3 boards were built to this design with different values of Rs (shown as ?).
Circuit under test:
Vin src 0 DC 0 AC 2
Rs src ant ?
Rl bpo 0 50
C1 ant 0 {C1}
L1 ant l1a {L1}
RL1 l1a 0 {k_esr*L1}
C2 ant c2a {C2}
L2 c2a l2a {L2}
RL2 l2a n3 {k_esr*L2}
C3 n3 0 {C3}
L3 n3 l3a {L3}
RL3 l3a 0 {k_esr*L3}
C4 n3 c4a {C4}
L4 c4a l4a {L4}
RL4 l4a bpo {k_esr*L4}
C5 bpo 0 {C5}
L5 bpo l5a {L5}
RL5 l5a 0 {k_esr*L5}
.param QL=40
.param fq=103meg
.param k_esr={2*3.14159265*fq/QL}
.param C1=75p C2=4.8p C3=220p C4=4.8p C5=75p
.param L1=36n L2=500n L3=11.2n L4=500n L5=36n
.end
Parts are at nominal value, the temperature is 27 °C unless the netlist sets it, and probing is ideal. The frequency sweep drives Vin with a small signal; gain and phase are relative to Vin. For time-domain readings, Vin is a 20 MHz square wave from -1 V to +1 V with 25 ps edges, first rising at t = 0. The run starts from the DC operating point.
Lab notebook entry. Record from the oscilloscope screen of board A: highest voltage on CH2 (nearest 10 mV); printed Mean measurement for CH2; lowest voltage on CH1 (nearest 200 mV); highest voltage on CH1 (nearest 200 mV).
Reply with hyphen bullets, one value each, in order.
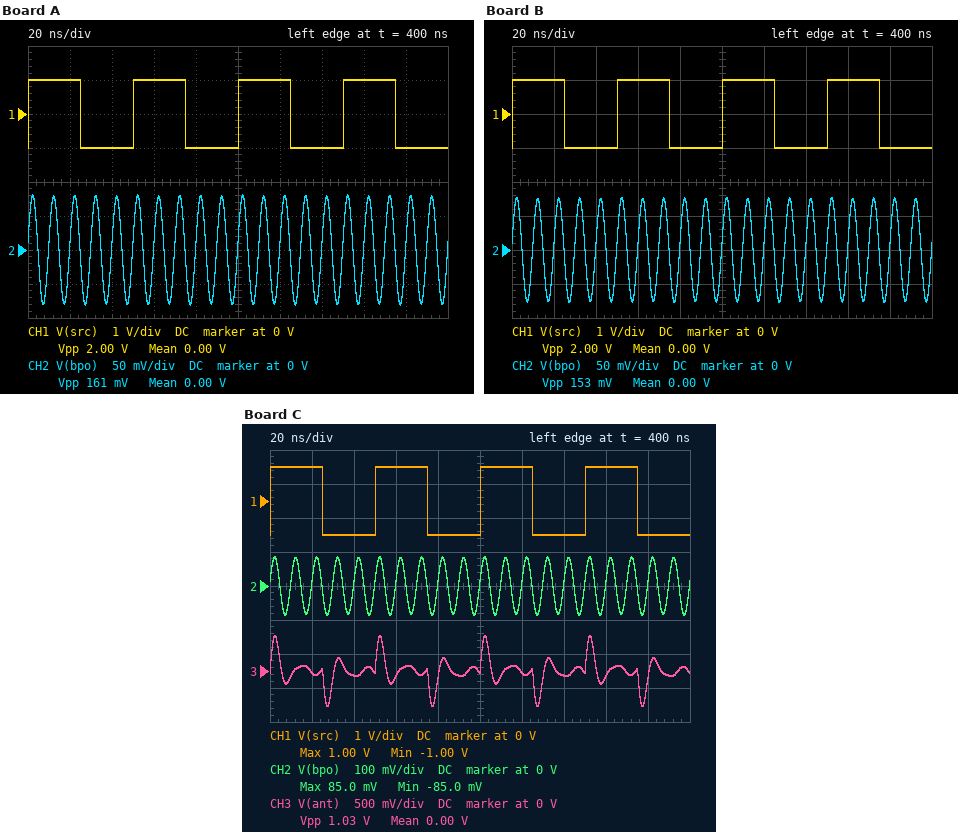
- 80 mV
- 0.00 V
- -1.0 V
- 1.0 V
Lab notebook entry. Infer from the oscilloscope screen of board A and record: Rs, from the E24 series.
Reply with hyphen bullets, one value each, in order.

- 62 Ω
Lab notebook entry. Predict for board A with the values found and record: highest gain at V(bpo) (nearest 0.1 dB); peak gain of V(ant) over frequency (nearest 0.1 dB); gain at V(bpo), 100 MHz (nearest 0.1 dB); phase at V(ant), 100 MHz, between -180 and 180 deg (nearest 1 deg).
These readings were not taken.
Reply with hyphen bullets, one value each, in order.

- -9.9 dB
- -1.5 dB
- -10.1 dB
- -16 deg
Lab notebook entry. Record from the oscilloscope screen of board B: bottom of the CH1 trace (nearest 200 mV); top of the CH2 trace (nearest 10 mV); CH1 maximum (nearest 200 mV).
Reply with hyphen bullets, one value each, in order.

- -1.0 V
- 80 mV
- 1.0 V
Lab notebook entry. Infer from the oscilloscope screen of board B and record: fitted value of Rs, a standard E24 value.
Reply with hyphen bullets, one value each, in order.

- 68 Ω
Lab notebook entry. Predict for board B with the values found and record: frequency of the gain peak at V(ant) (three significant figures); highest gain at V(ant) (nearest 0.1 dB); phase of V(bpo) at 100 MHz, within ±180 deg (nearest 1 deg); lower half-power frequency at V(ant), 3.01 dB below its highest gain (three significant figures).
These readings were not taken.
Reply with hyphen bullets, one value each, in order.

- 84.8 MHz
- -1.6 dB
- 13 deg
- 75.0 MHz
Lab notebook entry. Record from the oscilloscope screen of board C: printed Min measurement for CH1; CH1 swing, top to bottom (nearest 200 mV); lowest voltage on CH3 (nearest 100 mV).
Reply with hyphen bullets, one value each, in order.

- -1.00 V
- 2.0 V
- -500 mV
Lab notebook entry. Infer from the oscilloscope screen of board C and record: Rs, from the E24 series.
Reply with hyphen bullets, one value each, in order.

- 56 Ω
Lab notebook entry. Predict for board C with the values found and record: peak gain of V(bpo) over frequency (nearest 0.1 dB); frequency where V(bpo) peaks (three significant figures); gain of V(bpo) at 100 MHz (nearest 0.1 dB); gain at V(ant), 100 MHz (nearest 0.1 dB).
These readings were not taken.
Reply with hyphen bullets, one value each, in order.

- -9.4 dB
- 108 MHz
- -9.7 dB
- -5.7 dB
